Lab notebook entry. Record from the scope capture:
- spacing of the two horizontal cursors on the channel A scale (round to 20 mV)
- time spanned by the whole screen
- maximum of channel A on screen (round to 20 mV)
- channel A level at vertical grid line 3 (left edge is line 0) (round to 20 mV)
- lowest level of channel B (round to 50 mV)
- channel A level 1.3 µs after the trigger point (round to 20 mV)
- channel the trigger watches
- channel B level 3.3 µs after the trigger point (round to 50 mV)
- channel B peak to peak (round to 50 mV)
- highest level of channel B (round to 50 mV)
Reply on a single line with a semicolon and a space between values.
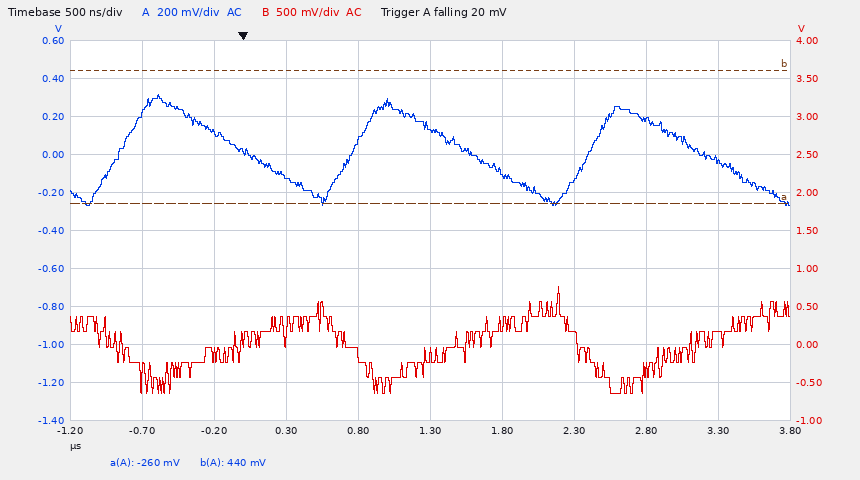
700 mV; 5 µs; 320 mV; -120 mV; -650 mV; 140 mV; channel A; 150 mV; 1.40 V; 750 mV
